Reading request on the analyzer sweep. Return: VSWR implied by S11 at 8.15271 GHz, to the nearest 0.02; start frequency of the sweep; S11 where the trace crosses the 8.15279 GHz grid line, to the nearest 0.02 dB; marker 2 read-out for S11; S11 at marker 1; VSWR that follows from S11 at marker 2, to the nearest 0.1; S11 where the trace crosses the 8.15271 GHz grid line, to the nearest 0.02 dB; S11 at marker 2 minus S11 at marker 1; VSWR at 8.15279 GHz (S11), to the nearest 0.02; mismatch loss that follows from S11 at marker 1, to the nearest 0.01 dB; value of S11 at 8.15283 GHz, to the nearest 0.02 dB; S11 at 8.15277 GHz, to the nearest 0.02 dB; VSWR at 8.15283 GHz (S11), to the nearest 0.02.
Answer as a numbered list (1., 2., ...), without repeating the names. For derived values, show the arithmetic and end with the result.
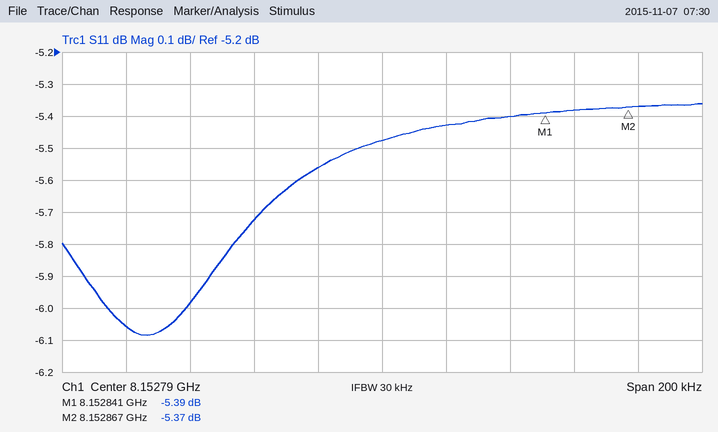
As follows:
1. |Γ| = 10^(-6.06/20) = 0.4977; VSWR = (1 + 0.4977)/(1 − 0.4977) ≈ 2.98
2. 8.15269 GHz
3. -5.48 dB
4. -5.37 dB
5. -5.39 dB
6. (1 + 0.5389)/(1 − 0.5389) ≈ 3.3
7. -6.06 dB
8. -5.37 − (-5.39) = 0.02 dB
9. |Γ| = 10^(-5.48/20) = 0.5321; VSWR = (1 + 0.5321)/(1 − 0.5321) ≈ 3.27, so 3.28 to the nearest 0.02
10. −10 log10(1 − 10^(-5.39/10)) ≈ 1.48 dB
11. -5.40 dB
12. -5.56 dB
13. |Γ| = 10^(-5.4/20) = 0.5370; VSWR = (1 + 0.5370)/(1 − 0.5370) ≈ 3.32
